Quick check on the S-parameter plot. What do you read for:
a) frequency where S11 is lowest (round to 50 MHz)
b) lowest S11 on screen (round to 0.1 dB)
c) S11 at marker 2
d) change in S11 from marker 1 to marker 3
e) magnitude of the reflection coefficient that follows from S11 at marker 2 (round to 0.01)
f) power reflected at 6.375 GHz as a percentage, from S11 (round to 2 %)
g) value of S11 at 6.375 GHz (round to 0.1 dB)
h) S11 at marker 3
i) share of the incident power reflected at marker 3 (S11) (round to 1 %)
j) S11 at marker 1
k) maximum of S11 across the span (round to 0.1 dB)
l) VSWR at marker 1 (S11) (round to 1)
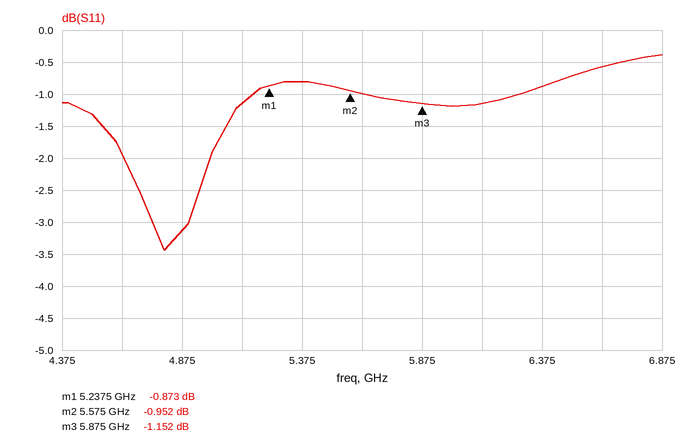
4.80 GHz
-3.4 dB
-0.952 dB
-0.279 dB
0.90
82 %
-0.9 dB
-1.152 dB
77 %
-0.873 dB
-0.4 dB
20
